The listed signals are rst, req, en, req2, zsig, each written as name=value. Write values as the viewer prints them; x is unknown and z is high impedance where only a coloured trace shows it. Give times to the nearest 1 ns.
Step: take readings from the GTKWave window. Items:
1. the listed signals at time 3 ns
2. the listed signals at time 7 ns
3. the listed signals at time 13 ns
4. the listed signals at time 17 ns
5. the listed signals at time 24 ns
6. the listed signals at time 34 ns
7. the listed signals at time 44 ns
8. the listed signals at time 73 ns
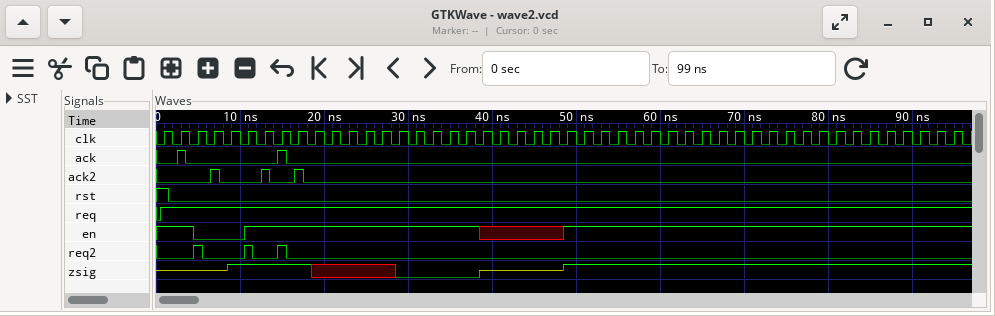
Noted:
rst=0, req=1, en=1, req2=0, zsig=z
rst=0, req=1, en=0, req2=0, zsig=z
rst=0, req=1, en=1, req2=0, zsig=1
rst=0, req=1, en=1, req2=0, zsig=1
rst=0, req=1, en=1, req2=0, zsig=x
rst=0, req=1, en=1, req2=0, zsig=0
rst=0, req=1, en=x, req2=0, zsig=z
rst=0, req=1, en=1, req2=0, zsig=1
